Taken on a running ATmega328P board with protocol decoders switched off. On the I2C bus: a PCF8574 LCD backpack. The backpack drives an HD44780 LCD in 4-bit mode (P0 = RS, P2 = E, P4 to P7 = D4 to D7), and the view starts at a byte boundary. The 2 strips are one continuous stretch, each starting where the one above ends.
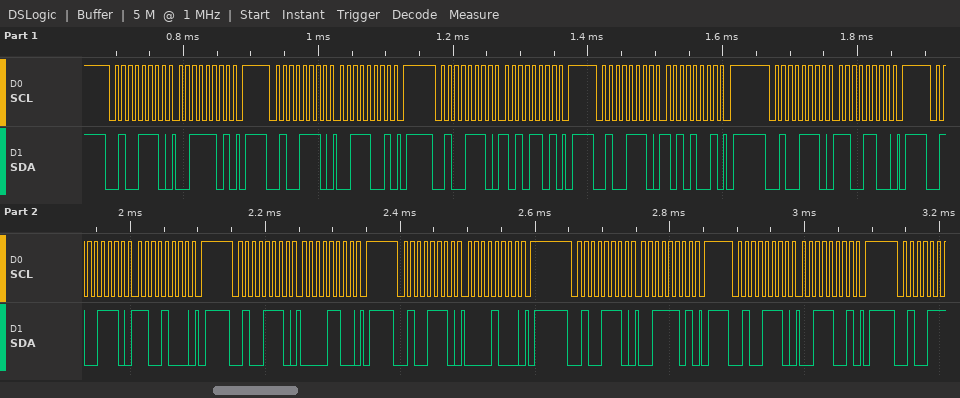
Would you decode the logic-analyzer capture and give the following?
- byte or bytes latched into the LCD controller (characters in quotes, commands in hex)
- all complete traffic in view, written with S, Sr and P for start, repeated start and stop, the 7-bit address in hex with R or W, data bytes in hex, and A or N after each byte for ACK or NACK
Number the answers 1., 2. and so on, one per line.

1. ':' 0xC0
2. S 27W A 3D A P S 27W A 39 A P S 27W A AD A P S 27W A A9 A P S 27W A CC A P S 27W A C8 A P S 27W A 0C A P S 27W A 08 A P S 27W A 3D A P S 27W A 39 A P
